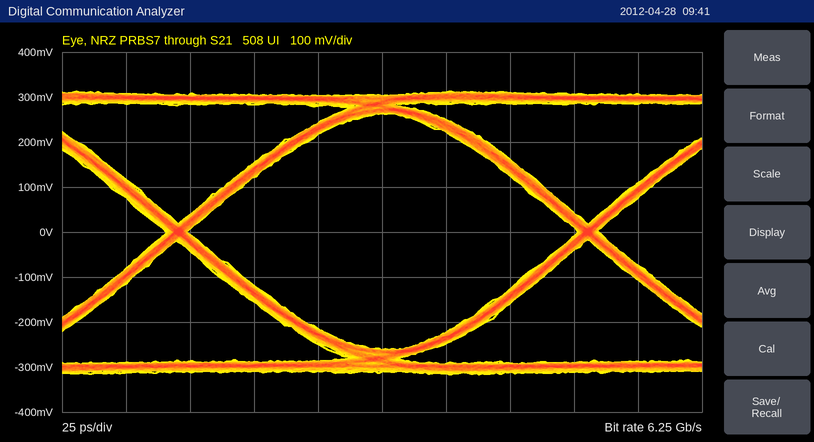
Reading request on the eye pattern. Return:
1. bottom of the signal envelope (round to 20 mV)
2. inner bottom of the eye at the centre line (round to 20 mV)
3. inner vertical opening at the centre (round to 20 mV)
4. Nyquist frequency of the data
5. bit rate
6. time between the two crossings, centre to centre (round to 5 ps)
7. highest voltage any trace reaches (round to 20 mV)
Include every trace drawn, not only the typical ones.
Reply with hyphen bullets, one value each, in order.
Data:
- -320 mV
- -260 mV
- 520 mV
- 3.125 GHz
- 6.25 Gb/s
- 160 ps
- 320 mV
